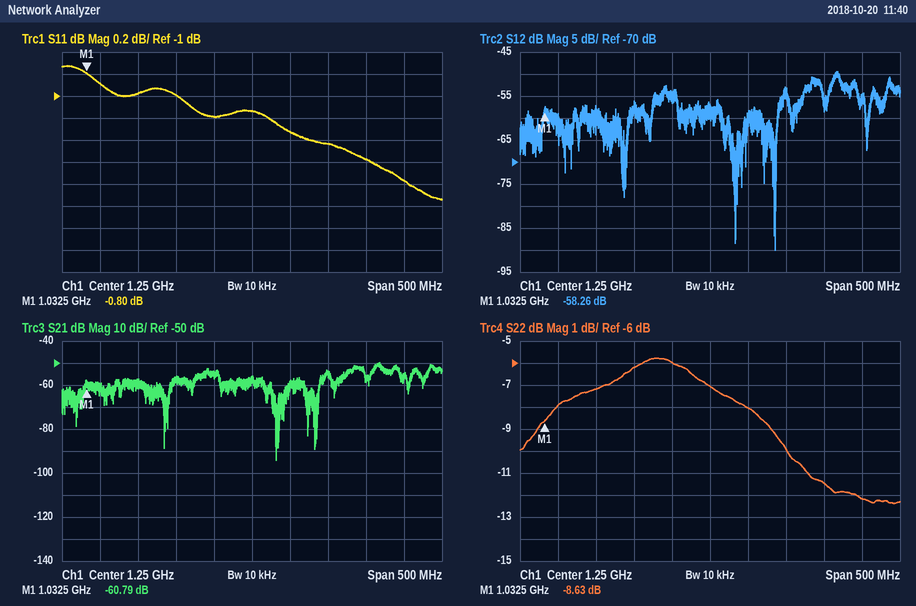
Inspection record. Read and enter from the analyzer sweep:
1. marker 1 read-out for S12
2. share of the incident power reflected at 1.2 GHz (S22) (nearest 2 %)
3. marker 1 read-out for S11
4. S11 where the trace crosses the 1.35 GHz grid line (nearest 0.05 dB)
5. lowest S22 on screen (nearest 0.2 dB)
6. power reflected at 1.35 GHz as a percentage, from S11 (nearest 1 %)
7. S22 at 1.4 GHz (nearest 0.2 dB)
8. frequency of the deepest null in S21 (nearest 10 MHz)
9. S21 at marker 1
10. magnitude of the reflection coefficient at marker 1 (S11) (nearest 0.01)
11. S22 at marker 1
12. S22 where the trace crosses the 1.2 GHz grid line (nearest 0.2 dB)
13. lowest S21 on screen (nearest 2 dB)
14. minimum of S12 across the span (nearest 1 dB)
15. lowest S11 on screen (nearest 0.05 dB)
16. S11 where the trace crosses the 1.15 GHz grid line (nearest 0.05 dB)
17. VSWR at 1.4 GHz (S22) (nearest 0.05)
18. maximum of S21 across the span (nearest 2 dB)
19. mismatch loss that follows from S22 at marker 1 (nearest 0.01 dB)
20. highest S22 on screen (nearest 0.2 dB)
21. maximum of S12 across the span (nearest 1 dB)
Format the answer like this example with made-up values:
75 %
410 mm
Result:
-58.26 dB
26 %
-0.80 dB
-1.45 dB
-12.4 dB
72 %
-11.4 dB
1.28 GHz
-60.79 dB
0.91
-8.63 dB
-6.0 dB
-94 dB
-90 dB
-1.95 dB
-1.00 dB
1.75
-50 dB
0.64 dB
-5.8 dB
-49 dB
